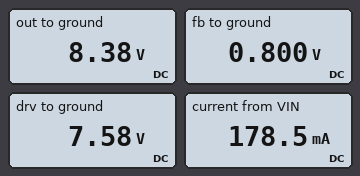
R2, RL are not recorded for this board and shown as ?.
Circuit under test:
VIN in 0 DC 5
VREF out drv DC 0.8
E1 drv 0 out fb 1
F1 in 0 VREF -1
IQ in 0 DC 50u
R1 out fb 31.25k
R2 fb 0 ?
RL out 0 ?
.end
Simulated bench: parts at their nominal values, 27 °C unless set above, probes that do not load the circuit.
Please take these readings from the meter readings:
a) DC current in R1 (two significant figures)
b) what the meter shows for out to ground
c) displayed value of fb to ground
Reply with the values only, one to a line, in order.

240 µA
8.38 V
0.800 V
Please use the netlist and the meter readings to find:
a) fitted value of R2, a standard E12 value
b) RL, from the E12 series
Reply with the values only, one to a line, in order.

3.3 kΩ
47 Ω
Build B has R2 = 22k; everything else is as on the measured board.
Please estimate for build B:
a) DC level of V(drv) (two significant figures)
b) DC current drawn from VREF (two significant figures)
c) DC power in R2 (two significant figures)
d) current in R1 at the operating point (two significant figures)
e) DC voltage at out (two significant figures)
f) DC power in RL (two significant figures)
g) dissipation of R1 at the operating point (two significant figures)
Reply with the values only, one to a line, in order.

1.1 V
41 mA
29 µW
36 µA
1.9 V
80 mW
41 µW
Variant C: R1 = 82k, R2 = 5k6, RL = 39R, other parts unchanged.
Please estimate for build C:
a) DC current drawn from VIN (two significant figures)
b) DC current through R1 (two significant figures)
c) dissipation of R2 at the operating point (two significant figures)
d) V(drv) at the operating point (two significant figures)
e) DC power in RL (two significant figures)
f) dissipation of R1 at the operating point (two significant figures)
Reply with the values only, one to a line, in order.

320 mA
140 µA
110 µW
12 V
4.0 W
1.7 mW
